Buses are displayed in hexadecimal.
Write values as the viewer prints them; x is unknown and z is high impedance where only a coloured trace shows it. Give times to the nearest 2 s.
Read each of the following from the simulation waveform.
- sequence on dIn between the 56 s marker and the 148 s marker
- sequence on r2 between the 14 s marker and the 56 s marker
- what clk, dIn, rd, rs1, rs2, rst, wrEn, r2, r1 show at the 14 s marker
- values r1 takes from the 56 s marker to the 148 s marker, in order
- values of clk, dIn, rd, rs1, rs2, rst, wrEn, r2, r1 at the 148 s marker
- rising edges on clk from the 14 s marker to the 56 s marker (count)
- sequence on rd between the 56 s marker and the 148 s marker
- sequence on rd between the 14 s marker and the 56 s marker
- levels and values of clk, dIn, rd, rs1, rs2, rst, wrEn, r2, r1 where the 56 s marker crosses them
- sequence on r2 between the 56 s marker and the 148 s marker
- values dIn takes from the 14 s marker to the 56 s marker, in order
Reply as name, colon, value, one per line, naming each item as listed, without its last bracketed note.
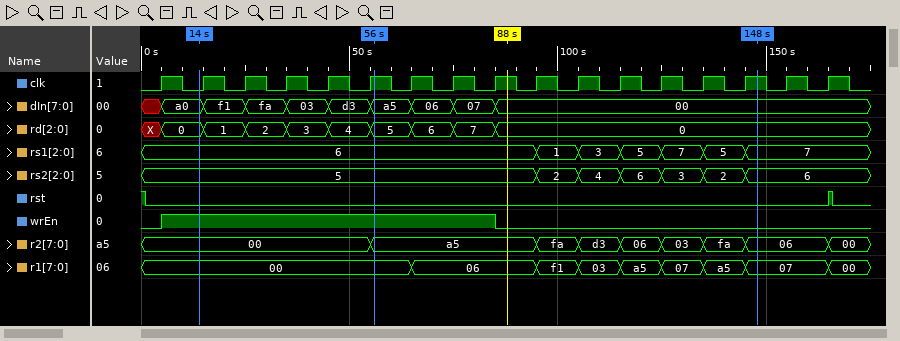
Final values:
sequence on dIn between the 56 s marker and the 148 s marker: a5, 06, 07, 00
sequence on r2 between the 14 s marker and the 56 s marker: 00, a5
what clk, dIn, rd, rs1, rs2, rst, wrEn, r2, r1 show at the 14 s marker: clk=0, dIn=a0, rd=0, rs1=6, rs2=5, rst=0, wrEn=1, r2=00, r1=00
values r1 takes from the 56 s marker to the 148 s marker, in order: 00, 06, f1, 03, a5, 07, a5, 07
values of clk, dIn, rd, rs1, rs2, rst, wrEn, r2, r1 at the 148 s marker: clk=1, dIn=00, rd=0, rs1=7, rs2=6, rst=0, wrEn=0, r2=06, r1=07
rising edges on clk from the 14 s marker to the 56 s marker: 5
sequence on rd between the 56 s marker and the 148 s marker: 5, 6, 7, 0
sequence on rd between the 14 s marker and the 56 s marker: 0, 1, 2, 3, 4, 5
levels and values of clk, dIn, rd, rs1, rs2, rst, wrEn, r2, r1 where the 56 s marker crosses them: clk=1, dIn=a5, rd=5, rs1=6, rs2=5, rst=0, wrEn=1, r2=a5, r1=00
sequence on r2 between the 56 s marker and the 148 s marker: a5, fa, d3, 06, 03, fa, 06
values dIn takes from the 14 s marker to the 56 s marker, in order: a0, f1, fa, 03, d3, a5
